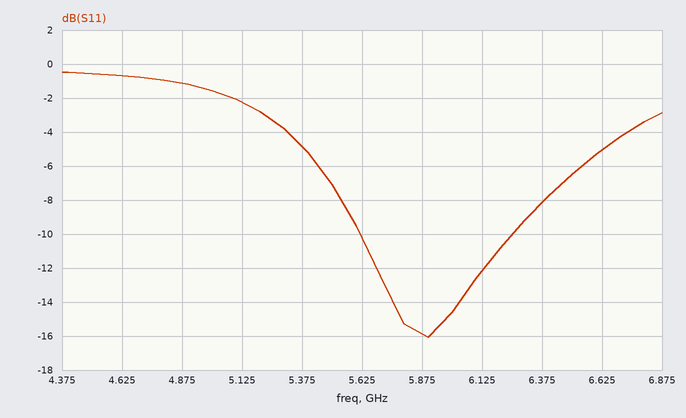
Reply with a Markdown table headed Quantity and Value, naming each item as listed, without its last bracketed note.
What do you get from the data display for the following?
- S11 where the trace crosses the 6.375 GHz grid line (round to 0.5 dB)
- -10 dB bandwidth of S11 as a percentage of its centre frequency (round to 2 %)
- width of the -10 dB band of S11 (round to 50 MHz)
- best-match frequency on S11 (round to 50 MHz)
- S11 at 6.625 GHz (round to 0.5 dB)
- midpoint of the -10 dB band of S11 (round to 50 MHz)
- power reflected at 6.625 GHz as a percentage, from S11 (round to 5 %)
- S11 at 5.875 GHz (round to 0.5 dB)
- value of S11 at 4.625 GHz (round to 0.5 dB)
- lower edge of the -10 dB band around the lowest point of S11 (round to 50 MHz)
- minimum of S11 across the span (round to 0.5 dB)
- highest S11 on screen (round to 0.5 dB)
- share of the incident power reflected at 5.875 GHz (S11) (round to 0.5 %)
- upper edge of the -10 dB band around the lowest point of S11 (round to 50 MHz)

| Quantity | Value |
|---|---|
| S11 where the trace crosses the 6.375 GHz grid line | -8.0 dB |
| -10 dB bandwidth of S11 as a percentage of its centre frequency | 10 % |
| width of the -10 dB band of S11 | 650 MHz |
| best-match frequency on S11 | 5.90 GHz |
| S11 at 6.625 GHz | -5.0 dB |
| midpoint of the -10 dB band of S11 | 5.95 GHz |
| power reflected at 6.625 GHz as a percentage, from S11 | 30 % |
| S11 at 5.875 GHz | -16.0 dB |
| value of S11 at 4.625 GHz | -0.5 dB |
| lower edge of the -10 dB band around the lowest point of S11 | 5.60 GHz |
| minimum of S11 across the span | -16.0 dB |
| highest S11 on screen | -0.5 dB |
| share of the incident power reflected at 5.875 GHz (S11) | 2.5 % |
| upper edge of the -10 dB band around the lowest point of S11 | 6.25 GHz |
